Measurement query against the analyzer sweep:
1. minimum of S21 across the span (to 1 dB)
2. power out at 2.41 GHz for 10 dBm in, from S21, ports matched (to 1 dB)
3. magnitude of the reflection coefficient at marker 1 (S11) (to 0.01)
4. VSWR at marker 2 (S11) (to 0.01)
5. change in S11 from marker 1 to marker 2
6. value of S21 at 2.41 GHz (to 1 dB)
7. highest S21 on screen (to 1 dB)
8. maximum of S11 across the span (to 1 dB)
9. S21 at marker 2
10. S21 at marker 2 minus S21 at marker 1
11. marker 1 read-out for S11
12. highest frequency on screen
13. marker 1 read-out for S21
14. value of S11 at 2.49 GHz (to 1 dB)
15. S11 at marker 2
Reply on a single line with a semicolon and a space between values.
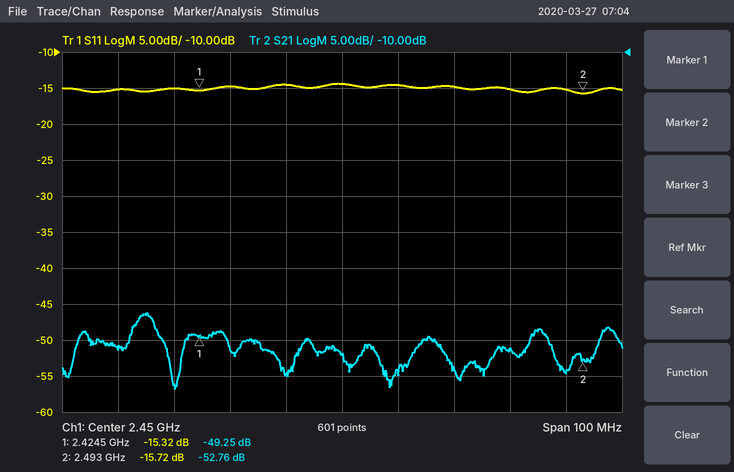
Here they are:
-57 dB; -41 dBm; 0.17; 1.39; -0.40 dB; -51 dB; -46 dB; -14 dB; -52.76 dB; -3.51 dB; -15.32 dB; 2.5 GHz; -49.25 dB; -15 dB; -15.72 dB
